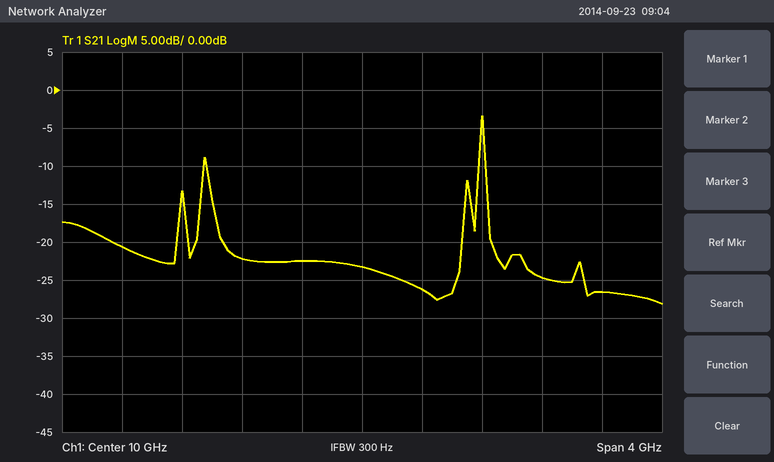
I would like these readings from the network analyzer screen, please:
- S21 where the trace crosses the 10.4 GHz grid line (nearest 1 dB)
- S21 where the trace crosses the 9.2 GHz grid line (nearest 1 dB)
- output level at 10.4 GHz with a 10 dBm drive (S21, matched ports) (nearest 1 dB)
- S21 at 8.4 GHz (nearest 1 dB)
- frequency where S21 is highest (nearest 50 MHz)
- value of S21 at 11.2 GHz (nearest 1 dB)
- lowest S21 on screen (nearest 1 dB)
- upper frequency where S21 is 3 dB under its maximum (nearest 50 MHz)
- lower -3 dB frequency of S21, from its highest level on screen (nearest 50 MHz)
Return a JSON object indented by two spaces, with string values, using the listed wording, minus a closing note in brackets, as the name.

{
  "S21 where the trace crosses the 10.4 GHz grid line": "-26 dB",
  "S21 where the trace crosses the 9.2 GHz grid line": "-22 dB",
  "output level at 10.4 GHz with a 10 dBm drive (S21, matched ports)": "-16 dBm",
  "S21 at 8.4 GHz": "-21 dB",
  "frequency where S21 is highest": "10.80 GHz",
  "value of S21 at 11.2 GHz": "-25 dB",
  "lowest S21 on screen": "-28 dB",
  "upper frequency where S21 is 3 dB under its maximum": "10.80 GHz",
  "lower -3 dB frequency of S21, from its highest level on screen": "10.80 GHz"
}
